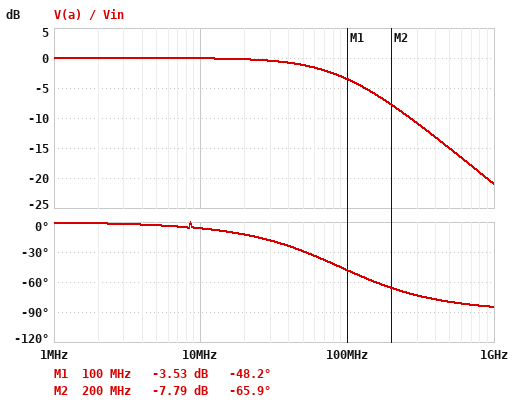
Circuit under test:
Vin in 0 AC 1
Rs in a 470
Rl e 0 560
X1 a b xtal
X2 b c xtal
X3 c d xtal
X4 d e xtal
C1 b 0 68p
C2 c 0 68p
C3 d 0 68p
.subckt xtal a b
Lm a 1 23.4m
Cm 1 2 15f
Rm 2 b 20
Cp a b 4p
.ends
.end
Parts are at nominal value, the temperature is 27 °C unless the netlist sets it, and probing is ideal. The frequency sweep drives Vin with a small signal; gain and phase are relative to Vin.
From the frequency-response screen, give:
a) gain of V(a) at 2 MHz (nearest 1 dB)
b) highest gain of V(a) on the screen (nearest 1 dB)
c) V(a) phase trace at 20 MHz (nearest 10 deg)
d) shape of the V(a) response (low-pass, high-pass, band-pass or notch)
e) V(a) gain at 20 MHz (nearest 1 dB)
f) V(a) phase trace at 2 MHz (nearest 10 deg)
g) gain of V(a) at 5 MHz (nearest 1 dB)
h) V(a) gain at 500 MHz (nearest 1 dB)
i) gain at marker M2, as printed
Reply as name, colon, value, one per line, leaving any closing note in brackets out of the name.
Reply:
gain of V(a) at 2 MHz: 0 dB
highest gain of V(a) on the screen: 0 dB
V(a) phase trace at 20 MHz: -10 deg
shape of the V(a) response: low-pass
V(a) gain at 20 MHz: 0 dB
V(a) phase trace at 2 MHz: 0 deg
gain of V(a) at 5 MHz: 0 dB
V(a) gain at 500 MHz: -15 dB
gain at marker M2, as printed: -7.79 dB
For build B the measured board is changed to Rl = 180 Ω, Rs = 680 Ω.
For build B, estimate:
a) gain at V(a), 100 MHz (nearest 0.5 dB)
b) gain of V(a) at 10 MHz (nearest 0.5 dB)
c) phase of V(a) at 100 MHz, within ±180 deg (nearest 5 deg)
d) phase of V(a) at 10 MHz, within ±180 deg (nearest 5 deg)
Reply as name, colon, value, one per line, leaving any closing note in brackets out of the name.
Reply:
gain at V(a), 100 MHz: -5.5 dB
gain of V(a) at 10 MHz: 0 dB
phase of V(a) at 100 MHz, within ±180 deg: -60 deg
phase of V(a) at 10 MHz, within ±180 deg: -10 deg
